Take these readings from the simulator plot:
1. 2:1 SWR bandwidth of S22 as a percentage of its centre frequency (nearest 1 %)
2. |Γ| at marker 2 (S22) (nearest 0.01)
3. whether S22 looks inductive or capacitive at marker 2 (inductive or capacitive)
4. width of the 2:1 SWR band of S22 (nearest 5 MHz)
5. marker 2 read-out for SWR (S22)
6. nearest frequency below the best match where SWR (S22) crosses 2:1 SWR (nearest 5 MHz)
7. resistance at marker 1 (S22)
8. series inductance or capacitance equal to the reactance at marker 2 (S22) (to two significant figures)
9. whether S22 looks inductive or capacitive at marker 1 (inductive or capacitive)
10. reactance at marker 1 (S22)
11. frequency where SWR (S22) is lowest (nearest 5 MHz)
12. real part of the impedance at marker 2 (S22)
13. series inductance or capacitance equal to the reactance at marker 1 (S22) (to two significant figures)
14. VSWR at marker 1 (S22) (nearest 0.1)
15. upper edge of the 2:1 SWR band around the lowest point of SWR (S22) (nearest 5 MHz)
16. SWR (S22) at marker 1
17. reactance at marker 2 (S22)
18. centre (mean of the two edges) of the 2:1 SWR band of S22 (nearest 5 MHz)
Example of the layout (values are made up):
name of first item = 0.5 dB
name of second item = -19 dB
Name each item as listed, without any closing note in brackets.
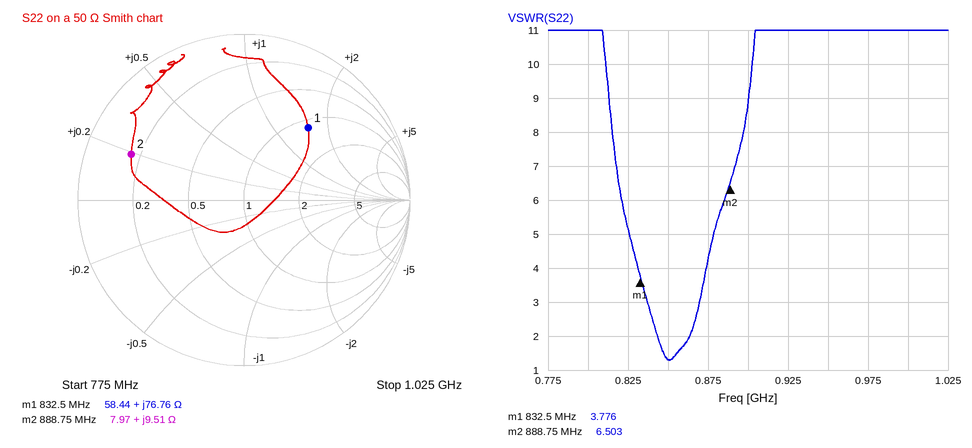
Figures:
2:1 SWR bandwidth of S22 as a percentage of its centre frequency = 2 %
|Γ| at marker 2 (S22) = 0.73
whether S22 looks inductive or capacitive at marker 2 = inductive
width of the 2:1 SWR band of S22 = 20 MHz
marker 2 read-out for SWR = 6.503
nearest frequency below the best match where SWR (S22) crosses 2:1 SWR = 845 MHz
resistance at marker 1 = 58.44 Ω
series inductance or capacitance equal to the reactance at marker 2 (S22) = 1.7 nH
whether S22 looks inductive or capacitive at marker 1 = inductive
reactance at marker 1 = +76.76 Ω
frequency where SWR (S22) is lowest = 850 MHz
real part of the impedance at marker 2 = 7.97 Ω
series inductance or capacitance equal to the reactance at marker 1 (S22) = 15 nH
VSWR at marker 1 (S22) = 3.8
upper edge of the 2:1 SWR band around the lowest point of SWR (S22) = 865 MHz
SWR (S22) at marker 1 = 3.776
reactance at marker 2 = +9.51 Ω
centre (mean of the two edges) of the 2:1 SWR band of S22 = 855 MHz
